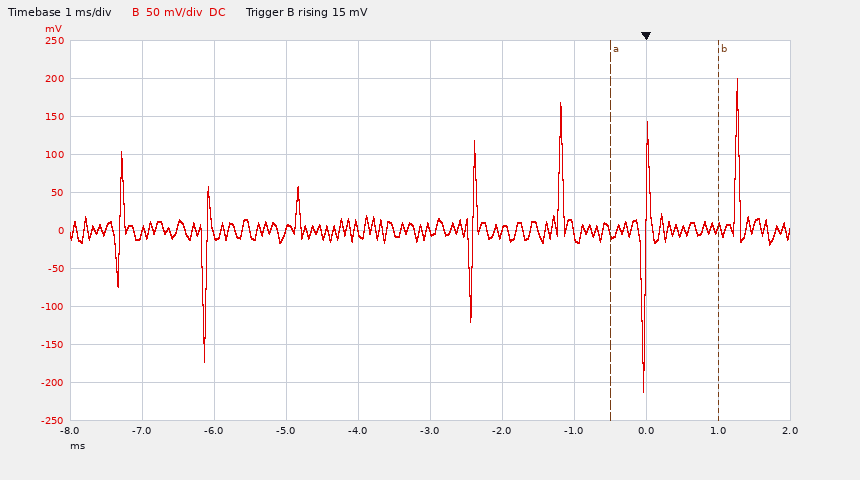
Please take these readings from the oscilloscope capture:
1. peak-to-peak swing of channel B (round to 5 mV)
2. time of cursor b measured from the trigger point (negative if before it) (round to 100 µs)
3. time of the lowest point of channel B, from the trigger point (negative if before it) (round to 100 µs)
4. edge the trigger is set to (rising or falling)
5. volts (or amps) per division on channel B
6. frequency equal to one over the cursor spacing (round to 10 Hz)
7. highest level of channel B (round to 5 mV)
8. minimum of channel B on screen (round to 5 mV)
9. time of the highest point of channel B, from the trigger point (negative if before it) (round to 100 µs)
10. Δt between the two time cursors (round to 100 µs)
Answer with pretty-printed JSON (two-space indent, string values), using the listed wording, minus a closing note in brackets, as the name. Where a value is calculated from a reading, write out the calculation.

{
  "peak-to-peak swing of channel B": "200 mV − (-210 mV) = 410 mV",
  "time of cursor b measured from the trigger point (negative if before it)": "+1.0 ms",
  "time of the lowest point of channel B, from the trigger point (negative if before it)": "0.0 ms",
  "edge the trigger is set to": "rising",
  "volts (or amps) per division on channel B": "50 mV",
  "frequency equal to one over the cursor spacing": "1 / 1.5 ms ≈ 670 Hz",
  "highest level of channel B": "200 mV",
  "minimum of channel B on screen": "-210 mV",
  "time of the highest point of channel B, from the trigger point (negative if before it)": "+1.3 ms",
  "Δt between the two time cursors": "1.5 ms"
}
